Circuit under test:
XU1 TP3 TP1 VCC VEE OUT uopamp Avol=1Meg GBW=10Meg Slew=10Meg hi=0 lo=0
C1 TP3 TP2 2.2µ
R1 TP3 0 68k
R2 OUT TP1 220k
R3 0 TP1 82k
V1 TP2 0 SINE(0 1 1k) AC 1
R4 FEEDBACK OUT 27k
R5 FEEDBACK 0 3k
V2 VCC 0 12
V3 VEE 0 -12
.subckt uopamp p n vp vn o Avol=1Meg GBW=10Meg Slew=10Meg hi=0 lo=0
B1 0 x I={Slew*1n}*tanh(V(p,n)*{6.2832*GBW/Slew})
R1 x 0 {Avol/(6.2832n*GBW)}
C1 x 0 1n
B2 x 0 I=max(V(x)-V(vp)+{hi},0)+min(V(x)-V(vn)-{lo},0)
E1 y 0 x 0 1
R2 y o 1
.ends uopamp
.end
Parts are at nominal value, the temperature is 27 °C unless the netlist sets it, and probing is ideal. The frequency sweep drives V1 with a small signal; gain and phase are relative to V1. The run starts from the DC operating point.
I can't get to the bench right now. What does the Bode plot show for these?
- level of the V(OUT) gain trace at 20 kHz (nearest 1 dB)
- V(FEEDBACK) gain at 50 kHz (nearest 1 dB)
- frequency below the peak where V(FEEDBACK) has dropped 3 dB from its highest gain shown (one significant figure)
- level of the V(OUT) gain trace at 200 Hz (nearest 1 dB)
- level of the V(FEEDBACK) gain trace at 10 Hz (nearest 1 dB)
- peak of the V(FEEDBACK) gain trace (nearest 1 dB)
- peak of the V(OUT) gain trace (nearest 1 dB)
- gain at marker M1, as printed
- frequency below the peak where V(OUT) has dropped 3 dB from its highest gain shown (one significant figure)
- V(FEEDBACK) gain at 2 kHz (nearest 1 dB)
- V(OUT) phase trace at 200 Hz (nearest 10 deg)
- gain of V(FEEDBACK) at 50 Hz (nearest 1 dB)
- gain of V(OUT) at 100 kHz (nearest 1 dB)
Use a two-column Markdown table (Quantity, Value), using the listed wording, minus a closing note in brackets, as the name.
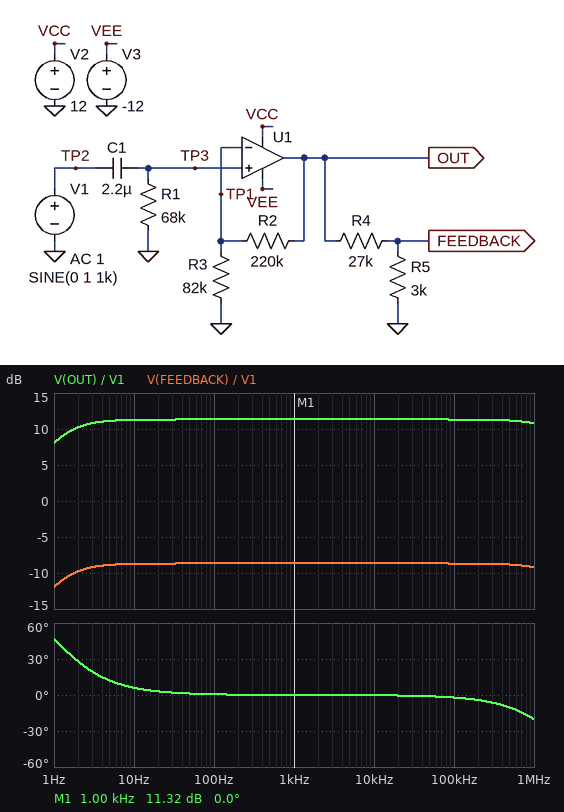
| Quantity | Value |
|---|---|
| level of the V(OUT) gain trace at 20 kHz | 11 dB |
| V(FEEDBACK) gain at 50 kHz | -9 dB |
| frequency below the peak where V(FEEDBACK) has dropped 3 dB from its highest gain shown | 1 Hz |
| level of the V(OUT) gain trace at 200 Hz | 11 dB |
| level of the V(FEEDBACK) gain trace at 10 Hz | -9 dB |
| peak of the V(FEEDBACK) gain trace | -9 dB |
| peak of the V(OUT) gain trace | 11 dB |
| gain at marker M1, as printed | 11.32 dB |
| frequency below the peak where V(OUT) has dropped 3 dB from its highest gain shown | 1 Hz |
| V(FEEDBACK) gain at 2 kHz | -9 dB |
| V(OUT) phase trace at 200 Hz | 0 deg |
| gain of V(FEEDBACK) at 50 Hz | -9 dB |
| gain of V(OUT) at 100 kHz | 11 dB |
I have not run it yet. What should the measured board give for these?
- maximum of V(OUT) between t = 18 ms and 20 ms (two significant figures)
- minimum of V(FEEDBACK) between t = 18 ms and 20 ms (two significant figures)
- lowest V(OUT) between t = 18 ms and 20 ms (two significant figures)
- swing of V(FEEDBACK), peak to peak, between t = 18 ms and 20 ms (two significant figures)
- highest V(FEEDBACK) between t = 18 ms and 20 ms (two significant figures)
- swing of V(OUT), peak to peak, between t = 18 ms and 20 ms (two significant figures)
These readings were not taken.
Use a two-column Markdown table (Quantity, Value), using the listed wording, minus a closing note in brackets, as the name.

| Quantity | Value |
|---|---|
| maximum of V(OUT) between t = 18 ms and 20 ms | 3.7 V |
| minimum of V(FEEDBACK) between t = 18 ms and 20 ms | -370 mV |
| lowest V(OUT) between t = 18 ms and 20 ms | -3.7 V |
| swing of V(FEEDBACK), peak to peak, between t = 18 ms and 20 ms | 740 mV |
| highest V(FEEDBACK) between t = 18 ms and 20 ms | 370 mV |
| swing of V(OUT), peak to peak, between t = 18 ms and 20 ms | 7.4 V |
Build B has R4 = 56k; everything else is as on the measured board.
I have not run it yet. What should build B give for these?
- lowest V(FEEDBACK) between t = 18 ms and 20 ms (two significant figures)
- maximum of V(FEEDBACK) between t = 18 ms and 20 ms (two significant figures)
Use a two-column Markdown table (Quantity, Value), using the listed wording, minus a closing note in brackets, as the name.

| Quantity | Value |
|---|---|
| lowest V(FEEDBACK) between t = 18 ms and 20 ms | -190 mV |
| maximum of V(FEEDBACK) between t = 18 ms and 20 ms | 190 mV |
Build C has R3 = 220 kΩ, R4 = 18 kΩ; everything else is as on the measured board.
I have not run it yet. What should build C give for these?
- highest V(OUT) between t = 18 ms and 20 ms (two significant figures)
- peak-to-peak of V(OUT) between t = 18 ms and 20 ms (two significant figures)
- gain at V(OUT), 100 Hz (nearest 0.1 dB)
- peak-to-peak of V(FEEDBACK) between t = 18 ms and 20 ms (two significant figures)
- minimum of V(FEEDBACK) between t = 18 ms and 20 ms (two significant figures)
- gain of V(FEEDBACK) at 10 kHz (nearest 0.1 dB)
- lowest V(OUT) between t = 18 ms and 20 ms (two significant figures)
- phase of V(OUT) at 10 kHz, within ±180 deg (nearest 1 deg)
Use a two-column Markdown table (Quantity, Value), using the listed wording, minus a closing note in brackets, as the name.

| Quantity | Value |
|---|---|
| highest V(OUT) between t = 18 ms and 20 ms | 2.0 V |
| peak-to-peak of V(OUT) between t = 18 ms and 20 ms | 4.0 V |
| gain at V(OUT), 100 Hz | 6.0 dB |
| peak-to-peak of V(FEEDBACK) between t = 18 ms and 20 ms | 570 mV |
| minimum of V(FEEDBACK) between t = 18 ms and 20 ms | -290 mV |
| gain of V(FEEDBACK) at 10 kHz | -10.9 dB |
| lowest V(OUT) between t = 18 ms and 20 ms | -2.0 V |
| phase of V(OUT) at 10 kHz, within ±180 deg | 0 deg |
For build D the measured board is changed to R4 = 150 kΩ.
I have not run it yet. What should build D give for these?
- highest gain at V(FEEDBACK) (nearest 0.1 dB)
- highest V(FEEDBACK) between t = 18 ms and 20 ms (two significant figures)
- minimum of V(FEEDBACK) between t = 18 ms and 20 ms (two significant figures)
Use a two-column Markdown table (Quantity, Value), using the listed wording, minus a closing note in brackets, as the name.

| Quantity | Value |
|---|---|
| highest gain at V(FEEDBACK) | -22.8 dB |
| highest V(FEEDBACK) between t = 18 ms and 20 ms | 72 mV |
| minimum of V(FEEDBACK) between t = 18 ms and 20 ms | -72 mV |
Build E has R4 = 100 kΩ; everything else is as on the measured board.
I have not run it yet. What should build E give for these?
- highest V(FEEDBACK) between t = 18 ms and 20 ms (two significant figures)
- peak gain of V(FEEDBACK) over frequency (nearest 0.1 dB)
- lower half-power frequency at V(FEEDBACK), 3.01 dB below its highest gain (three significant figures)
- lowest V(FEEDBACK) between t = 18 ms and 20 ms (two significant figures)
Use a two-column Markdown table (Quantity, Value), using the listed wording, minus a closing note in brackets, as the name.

| Quantity | Value |
|---|---|
| highest V(FEEDBACK) between t = 18 ms and 20 ms | 110 mV |
| peak gain of V(FEEDBACK) over frequency | -19.4 dB |
| lower half-power frequency at V(FEEDBACK), 3.01 dB below its highest gain | 1.06 Hz |
| lowest V(FEEDBACK) between t = 18 ms and 20 ms | -110 mV |
